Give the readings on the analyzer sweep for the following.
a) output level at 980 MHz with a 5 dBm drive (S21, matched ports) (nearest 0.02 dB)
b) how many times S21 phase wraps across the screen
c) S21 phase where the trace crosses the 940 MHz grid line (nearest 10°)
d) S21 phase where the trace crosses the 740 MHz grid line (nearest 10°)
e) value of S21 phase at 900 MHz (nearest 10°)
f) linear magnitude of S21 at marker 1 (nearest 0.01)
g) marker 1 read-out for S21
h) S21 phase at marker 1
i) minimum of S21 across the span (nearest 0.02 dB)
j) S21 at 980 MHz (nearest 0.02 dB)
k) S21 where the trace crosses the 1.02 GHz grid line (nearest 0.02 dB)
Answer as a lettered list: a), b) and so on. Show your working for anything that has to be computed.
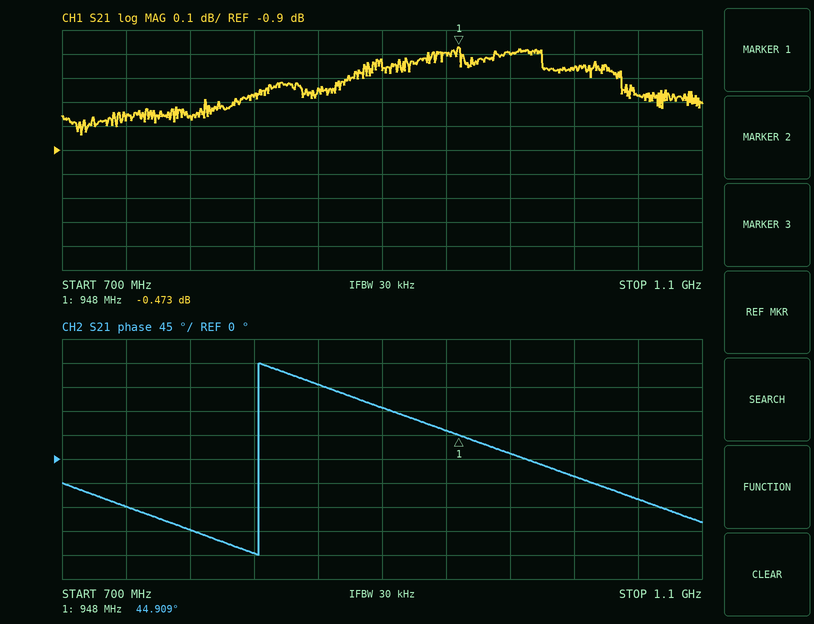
a) 5 dBm + (-0.50 dB) = 4.50 dBm
b) 1
c) 50°
d) -90°
e) 100°
f) 10^(-0.473/20) ≈ 0.95
g) -0.473 dB
h) 44.909°
i) -0.84 dB
j) -0.50 dB
k) -0.56 dB
